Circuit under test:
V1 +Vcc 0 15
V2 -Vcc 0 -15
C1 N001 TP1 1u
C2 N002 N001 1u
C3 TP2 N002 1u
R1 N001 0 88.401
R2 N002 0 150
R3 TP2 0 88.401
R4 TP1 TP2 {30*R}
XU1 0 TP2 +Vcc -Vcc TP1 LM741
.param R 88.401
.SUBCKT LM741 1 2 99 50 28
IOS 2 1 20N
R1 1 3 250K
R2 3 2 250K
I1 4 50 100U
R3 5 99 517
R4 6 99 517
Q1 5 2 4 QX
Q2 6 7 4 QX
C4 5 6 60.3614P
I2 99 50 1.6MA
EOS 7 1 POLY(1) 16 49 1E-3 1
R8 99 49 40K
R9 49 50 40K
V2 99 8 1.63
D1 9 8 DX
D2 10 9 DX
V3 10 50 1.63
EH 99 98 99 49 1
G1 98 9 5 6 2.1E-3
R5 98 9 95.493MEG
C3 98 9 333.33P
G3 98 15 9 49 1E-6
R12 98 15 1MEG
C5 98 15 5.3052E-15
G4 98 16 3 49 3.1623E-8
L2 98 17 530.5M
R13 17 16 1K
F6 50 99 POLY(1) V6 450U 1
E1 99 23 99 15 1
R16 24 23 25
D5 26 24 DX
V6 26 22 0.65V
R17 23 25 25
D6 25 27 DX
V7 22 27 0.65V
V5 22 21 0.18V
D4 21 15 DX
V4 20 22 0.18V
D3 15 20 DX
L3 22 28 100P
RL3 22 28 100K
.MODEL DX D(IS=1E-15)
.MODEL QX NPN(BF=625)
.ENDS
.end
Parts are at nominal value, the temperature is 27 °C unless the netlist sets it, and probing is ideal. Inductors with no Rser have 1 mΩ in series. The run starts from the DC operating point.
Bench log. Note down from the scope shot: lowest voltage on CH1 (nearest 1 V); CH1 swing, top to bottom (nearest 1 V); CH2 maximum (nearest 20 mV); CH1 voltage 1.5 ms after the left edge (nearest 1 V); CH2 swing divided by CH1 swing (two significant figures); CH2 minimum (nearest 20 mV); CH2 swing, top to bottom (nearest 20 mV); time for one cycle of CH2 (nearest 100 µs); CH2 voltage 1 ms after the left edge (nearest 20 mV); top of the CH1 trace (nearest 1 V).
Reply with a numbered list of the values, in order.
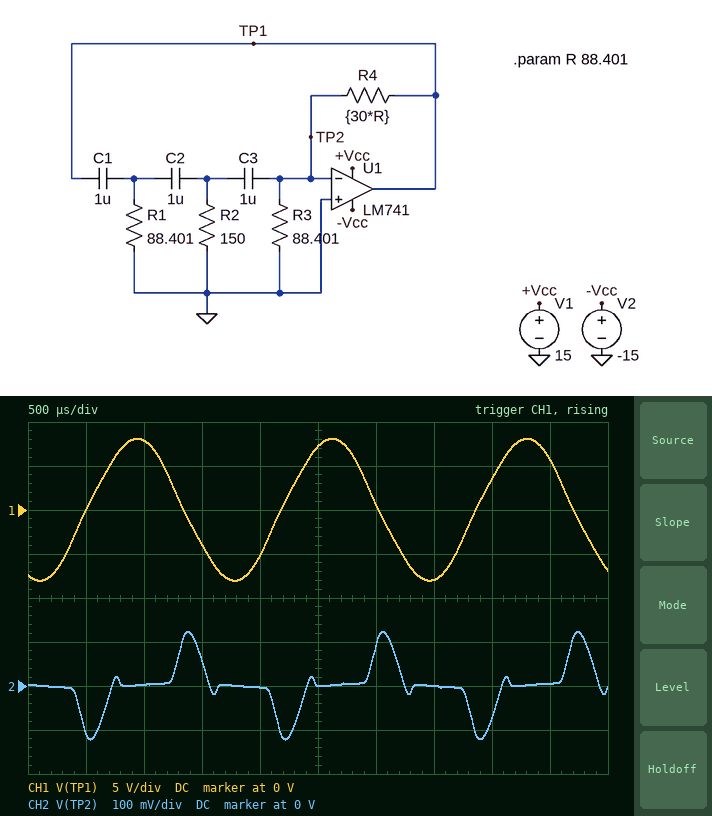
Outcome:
1. -8 V
2. 16 V
3. 120 mV
4. -4 V
5. 0.015
6. -120 mV
7. 240 mV
8. 1.7 ms
9. 0 V
10. 8 V
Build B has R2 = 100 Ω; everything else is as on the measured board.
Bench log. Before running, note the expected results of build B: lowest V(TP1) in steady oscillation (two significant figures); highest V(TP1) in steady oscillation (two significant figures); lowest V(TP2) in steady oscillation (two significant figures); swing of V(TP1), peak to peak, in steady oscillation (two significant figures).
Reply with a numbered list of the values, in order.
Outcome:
1. -7.6 V
2. 7.7 V
3. -140 mV
4. 15 V
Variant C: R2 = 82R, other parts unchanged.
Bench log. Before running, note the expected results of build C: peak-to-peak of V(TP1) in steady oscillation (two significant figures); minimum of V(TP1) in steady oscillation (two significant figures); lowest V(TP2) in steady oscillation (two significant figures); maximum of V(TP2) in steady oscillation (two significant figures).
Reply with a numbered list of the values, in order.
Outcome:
1. 15 V
2. -7.4 V
3. -150 mV
4. 150 mV
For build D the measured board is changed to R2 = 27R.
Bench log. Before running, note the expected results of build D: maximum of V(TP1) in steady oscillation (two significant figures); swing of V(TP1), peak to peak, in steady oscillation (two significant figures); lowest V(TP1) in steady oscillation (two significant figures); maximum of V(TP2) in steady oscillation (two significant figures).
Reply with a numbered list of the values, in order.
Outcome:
1. 6.1 V
2. 12 V
3. -6.0 V
4. 130 mV
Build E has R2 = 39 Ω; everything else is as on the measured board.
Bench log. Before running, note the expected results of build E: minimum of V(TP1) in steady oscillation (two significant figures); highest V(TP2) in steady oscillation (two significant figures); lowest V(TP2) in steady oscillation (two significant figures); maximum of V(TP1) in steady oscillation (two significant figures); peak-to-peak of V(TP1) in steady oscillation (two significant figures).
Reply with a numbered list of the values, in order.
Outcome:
1. -6.5 V
2. 140 mV
3. -140 mV
4. 6.5 V
5. 13 V
